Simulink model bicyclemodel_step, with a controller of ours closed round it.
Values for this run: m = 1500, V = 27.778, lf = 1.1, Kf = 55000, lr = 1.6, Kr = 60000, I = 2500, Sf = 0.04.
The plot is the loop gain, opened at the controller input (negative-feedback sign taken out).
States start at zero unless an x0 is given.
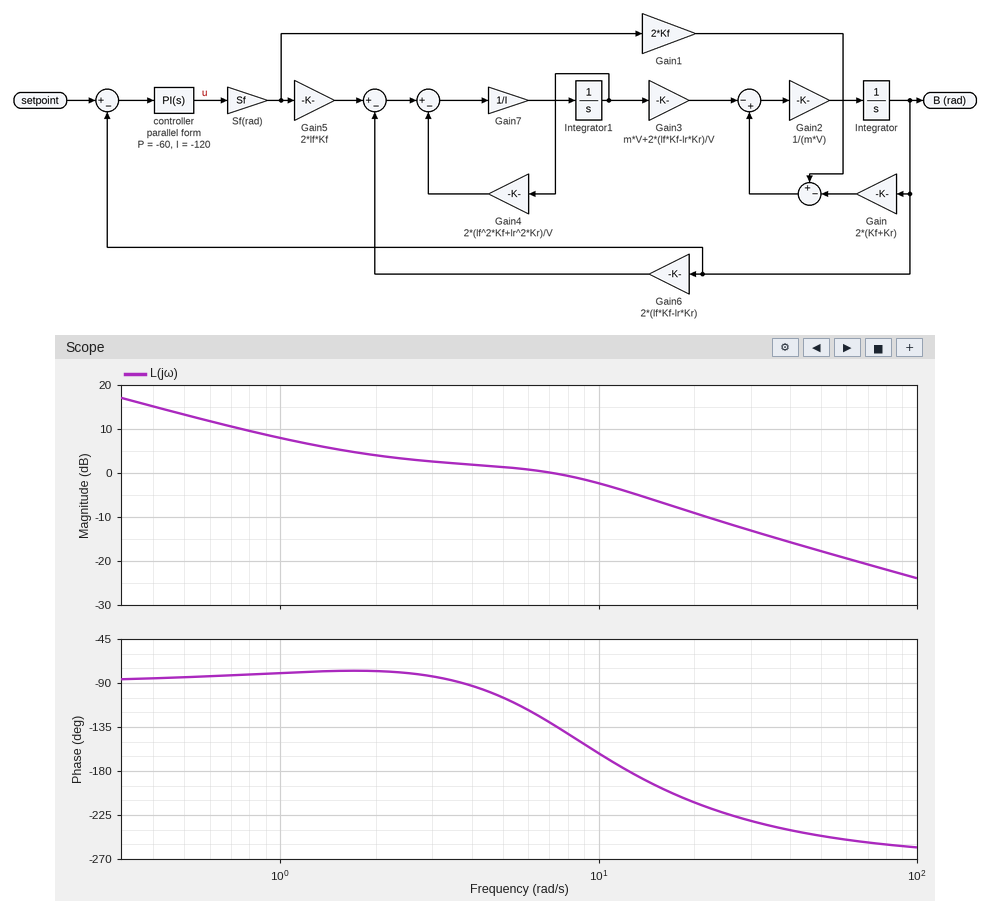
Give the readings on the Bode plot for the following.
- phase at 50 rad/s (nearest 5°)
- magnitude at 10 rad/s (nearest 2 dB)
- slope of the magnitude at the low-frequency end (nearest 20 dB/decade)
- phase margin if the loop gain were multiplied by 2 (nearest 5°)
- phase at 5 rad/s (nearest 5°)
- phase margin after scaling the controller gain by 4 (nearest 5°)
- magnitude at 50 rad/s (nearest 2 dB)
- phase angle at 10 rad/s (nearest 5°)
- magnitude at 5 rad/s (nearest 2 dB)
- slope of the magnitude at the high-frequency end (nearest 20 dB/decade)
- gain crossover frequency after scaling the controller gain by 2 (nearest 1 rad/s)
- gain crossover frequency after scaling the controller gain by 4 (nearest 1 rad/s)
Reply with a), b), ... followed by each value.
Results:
a) -245°
b) -2 dB
c) -20 dB/decade
d) -15°
e) -105°
f) -45°
g) -18 dB
h) -160°
i) 2 dB
j) -20 dB/decade
k) 15 rad/s
l) 27 rad/s
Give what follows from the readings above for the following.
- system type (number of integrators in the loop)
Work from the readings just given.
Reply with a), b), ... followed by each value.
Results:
a) 1
